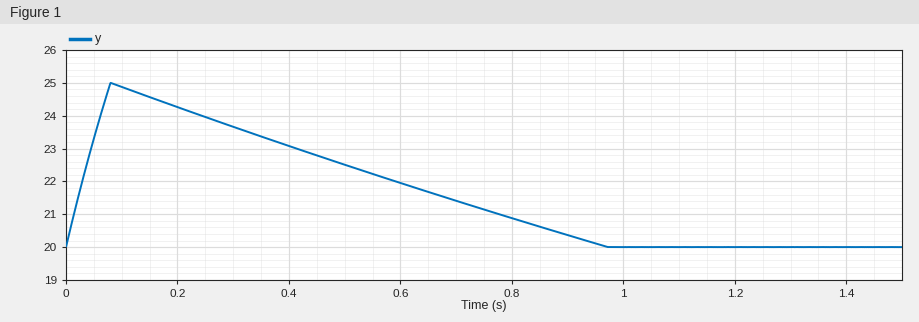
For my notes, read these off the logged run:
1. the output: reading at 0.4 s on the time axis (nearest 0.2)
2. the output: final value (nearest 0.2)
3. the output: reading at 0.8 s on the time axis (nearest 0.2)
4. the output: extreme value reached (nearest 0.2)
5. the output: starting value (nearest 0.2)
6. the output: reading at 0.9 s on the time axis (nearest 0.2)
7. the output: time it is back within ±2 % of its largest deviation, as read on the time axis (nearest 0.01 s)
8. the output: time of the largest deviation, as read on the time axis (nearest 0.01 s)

23.0
20.0
20.8
25.0
20.0
20.4
0.95 s
0.08 s
